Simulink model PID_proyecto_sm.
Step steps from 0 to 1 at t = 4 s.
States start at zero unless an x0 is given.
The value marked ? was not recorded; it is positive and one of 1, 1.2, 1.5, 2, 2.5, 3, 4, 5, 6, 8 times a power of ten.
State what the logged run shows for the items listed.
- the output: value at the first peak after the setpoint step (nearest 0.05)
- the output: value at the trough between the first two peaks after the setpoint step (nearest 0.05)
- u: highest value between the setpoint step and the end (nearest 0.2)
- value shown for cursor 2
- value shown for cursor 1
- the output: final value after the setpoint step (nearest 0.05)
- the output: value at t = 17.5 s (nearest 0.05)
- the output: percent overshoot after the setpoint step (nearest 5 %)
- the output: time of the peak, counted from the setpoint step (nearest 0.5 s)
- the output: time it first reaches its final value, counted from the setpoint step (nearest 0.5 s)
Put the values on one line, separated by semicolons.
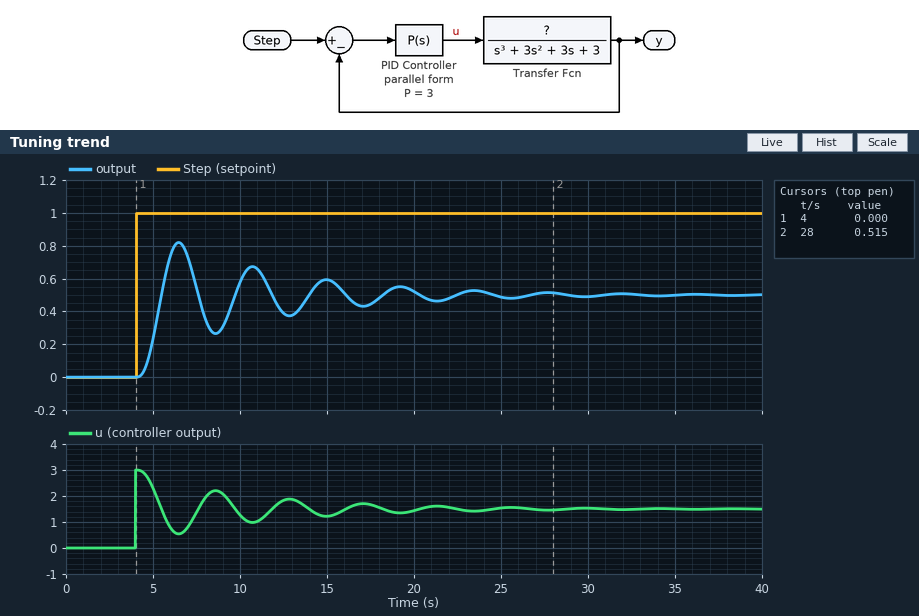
0.80; 0.25; 3.0; 0.515; 0.000; 0.50; 0.45; 65 %; 2.5 s; 1.5 s
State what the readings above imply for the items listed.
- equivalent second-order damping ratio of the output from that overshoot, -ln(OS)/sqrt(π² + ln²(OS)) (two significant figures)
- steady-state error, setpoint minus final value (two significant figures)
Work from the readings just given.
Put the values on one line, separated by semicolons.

0.14; 0.50
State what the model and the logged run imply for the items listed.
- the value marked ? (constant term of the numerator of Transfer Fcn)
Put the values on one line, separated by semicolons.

1
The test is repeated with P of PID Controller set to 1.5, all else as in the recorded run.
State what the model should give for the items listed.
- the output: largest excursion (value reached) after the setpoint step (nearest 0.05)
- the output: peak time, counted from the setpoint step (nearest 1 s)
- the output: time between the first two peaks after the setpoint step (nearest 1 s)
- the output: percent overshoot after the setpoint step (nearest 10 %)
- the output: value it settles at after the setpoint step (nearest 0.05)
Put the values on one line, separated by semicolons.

0.50; 3 s; 5 s; 50 %; 0.35
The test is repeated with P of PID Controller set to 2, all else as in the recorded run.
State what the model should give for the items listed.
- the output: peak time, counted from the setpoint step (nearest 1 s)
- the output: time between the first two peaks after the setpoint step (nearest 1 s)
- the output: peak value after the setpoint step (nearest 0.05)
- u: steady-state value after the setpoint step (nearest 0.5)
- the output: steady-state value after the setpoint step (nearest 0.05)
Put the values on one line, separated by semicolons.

3 s; 5 s; 0.60; 1.0; 0.40
